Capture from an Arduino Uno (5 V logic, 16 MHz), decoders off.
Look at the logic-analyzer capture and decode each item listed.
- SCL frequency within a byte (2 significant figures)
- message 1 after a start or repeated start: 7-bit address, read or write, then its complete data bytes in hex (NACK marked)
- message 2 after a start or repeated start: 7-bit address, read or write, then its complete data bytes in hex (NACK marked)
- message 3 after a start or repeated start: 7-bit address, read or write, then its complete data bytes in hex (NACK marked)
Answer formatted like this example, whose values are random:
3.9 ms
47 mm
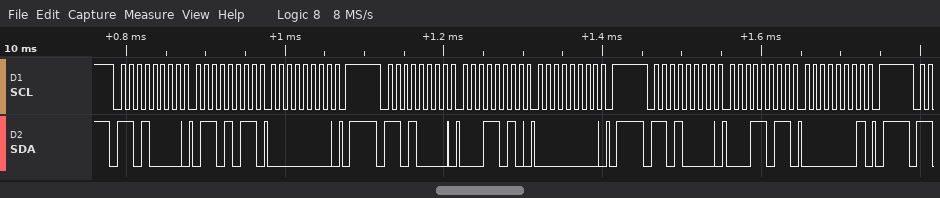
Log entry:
100 kHz
0x68 write: 6B 00
0x68 write: 1A 00
0x68 write: 1B 01
